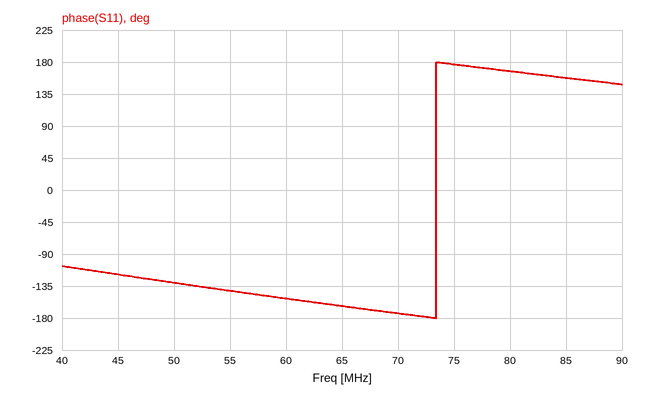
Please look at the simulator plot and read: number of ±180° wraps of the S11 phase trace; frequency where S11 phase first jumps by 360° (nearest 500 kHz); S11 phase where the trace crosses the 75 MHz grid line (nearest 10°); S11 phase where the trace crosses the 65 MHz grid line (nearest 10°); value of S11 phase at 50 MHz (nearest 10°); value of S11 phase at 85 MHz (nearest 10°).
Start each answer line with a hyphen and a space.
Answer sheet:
- 1
- 73.5 MHz
- 180°
- -160°
- -130°
- 160°
